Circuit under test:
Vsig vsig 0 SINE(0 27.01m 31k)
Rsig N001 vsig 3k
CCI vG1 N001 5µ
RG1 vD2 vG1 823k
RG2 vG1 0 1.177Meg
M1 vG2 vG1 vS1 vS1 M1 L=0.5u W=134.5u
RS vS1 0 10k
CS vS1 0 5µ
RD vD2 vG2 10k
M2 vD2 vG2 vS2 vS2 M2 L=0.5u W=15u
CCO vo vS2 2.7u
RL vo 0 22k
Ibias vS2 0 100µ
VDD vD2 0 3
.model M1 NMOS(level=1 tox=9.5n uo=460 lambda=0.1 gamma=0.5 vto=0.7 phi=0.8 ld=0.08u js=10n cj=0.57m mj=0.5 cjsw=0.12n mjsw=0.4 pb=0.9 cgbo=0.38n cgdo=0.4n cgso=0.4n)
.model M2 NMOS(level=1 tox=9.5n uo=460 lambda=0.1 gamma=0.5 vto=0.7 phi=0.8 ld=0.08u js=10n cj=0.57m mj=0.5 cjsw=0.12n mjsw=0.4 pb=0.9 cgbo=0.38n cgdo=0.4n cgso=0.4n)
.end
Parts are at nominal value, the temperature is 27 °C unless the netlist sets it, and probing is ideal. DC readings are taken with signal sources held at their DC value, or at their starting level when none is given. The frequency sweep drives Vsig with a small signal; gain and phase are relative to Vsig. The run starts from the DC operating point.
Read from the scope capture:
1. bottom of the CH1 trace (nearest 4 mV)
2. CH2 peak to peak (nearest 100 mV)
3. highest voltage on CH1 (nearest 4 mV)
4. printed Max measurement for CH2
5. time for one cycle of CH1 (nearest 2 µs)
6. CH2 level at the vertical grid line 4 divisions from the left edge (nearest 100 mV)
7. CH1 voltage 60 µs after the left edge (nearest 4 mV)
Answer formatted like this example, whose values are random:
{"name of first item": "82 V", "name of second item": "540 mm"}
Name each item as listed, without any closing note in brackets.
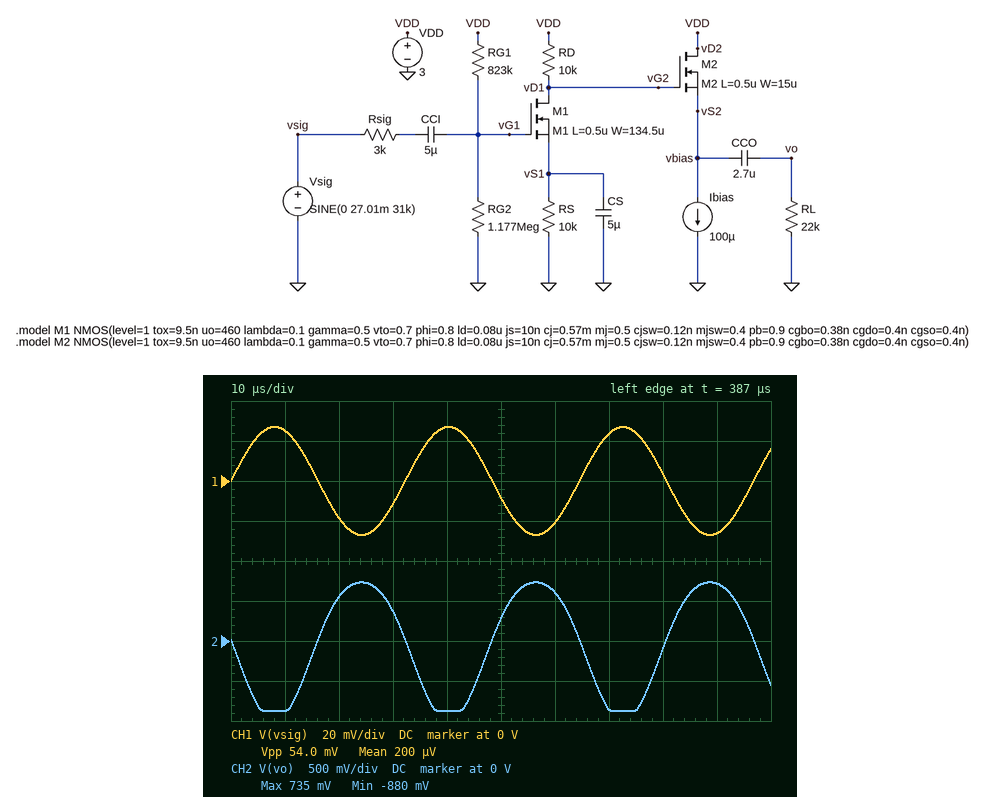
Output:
{"bottom of the CH1 trace": "-28 mV", "CH2 peak to peak": "1.6 V", "highest voltage on CH1": "28 mV", "printed Max measurement for CH2": "735 mV", "time for one cycle of CH1": "32 µs", "CH2 level at the vertical grid line 4 divisions from the left edge": "-900 mV", "CH1 voltage 60 µs after the left edge": "-20 mV"}
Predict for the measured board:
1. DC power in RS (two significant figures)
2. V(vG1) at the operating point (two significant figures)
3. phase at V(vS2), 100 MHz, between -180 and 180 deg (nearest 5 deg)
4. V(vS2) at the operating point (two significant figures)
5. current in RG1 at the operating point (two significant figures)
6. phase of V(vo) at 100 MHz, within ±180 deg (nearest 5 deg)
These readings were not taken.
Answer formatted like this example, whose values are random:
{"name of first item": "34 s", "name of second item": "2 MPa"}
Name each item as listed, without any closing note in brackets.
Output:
{"DC power in RS": "100 µW", "V(vG1) at the operating point": "1.8 V", "phase at V(vS2), 100 MHz, between -180 and 180 deg": "100 deg", "V(vS2) at the operating point": "1.1 V", "current in RG1 at the operating point": "1.5 µA", "phase of V(vo) at 100 MHz, within ±180 deg": "100 deg"}
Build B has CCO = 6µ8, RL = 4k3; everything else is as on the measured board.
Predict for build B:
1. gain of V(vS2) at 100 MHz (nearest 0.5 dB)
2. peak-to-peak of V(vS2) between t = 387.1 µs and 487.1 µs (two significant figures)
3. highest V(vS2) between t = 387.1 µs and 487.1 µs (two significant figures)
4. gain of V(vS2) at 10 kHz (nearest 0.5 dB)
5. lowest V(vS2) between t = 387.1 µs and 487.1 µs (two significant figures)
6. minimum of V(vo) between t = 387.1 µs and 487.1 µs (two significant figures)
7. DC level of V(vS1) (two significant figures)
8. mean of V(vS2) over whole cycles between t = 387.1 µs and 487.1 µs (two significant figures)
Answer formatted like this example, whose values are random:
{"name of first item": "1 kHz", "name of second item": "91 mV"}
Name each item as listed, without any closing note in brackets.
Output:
{"gain of V(vS2) at 100 MHz": "16.5 dB", "peak-to-peak of V(vS2) between t = 387.1 µs and 487.1 µs": "1.1 V", "highest V(vS2) between t = 387.1 µs and 487.1 µs": "1.8 V", "gain of V(vS2) at 10 kHz": "29.5 dB", "lowest V(vS2) between t = 387.1 µs and 487.1 µs": "710 mV", "minimum of V(vo) between t = 387.1 µs and 487.1 µs": "-430 mV", "DC level of V(vS1)": "1.0 V", "mean of V(vS2) over whole cycles between t = 387.1 µs and 487.1 µs": "1.2 V"}
